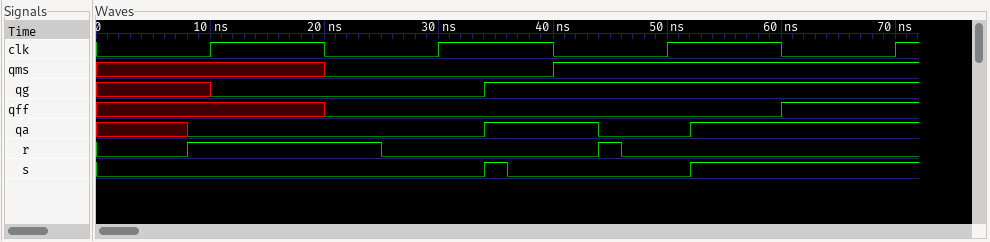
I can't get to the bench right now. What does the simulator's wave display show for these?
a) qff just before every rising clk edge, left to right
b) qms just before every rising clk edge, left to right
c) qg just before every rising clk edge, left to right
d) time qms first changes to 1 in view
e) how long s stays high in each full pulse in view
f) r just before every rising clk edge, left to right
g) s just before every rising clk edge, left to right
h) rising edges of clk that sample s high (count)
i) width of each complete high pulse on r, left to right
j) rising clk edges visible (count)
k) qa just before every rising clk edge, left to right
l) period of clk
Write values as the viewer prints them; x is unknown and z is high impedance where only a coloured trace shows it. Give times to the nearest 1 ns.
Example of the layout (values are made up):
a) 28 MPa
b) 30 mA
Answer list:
a) x 0 0 1
b) x 0 1 1
c) x 0 1 1
d) 40 ns
e) 2 ns
f) 1 0 0 0
g) 0 0 0 1
h) 1
i) 17 ns, 2 ns
j) 4
k) 0 0 0 1
l) 20 ns
